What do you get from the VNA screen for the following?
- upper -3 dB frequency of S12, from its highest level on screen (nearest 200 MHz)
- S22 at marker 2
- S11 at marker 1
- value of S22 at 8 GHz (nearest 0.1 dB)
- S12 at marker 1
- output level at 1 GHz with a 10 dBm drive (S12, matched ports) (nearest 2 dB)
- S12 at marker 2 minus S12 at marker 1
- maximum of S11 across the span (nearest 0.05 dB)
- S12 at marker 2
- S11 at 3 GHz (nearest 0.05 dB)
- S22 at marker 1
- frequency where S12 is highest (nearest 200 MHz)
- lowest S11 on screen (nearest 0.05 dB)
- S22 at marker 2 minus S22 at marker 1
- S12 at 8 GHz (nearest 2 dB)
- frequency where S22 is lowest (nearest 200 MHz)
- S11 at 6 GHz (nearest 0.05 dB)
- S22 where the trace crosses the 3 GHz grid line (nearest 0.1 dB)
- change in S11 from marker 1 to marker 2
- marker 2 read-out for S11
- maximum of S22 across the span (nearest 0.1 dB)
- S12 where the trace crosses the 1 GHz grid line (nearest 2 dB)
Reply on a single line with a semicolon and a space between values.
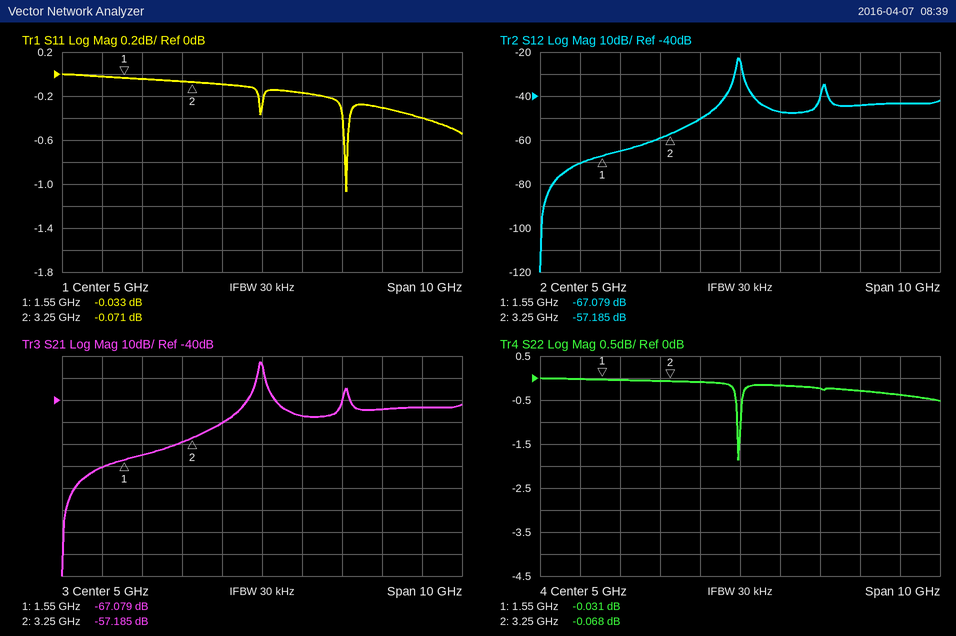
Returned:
5.0 GHz; -0.068 dB; -0.033 dB; -0.3 dB; -67.079 dB; -60 dBm; 9.894 dB; 0.00 dB; -57.185 dB; -0.05 dB; -0.031 dB; 5.0 GHz; -1.05 dB; -0.037 dB; -44 dB; 5.0 GHz; -0.15 dB; -0.1 dB; -0.038 dB; -0.071 dB; 0.0 dB; -70 dB
